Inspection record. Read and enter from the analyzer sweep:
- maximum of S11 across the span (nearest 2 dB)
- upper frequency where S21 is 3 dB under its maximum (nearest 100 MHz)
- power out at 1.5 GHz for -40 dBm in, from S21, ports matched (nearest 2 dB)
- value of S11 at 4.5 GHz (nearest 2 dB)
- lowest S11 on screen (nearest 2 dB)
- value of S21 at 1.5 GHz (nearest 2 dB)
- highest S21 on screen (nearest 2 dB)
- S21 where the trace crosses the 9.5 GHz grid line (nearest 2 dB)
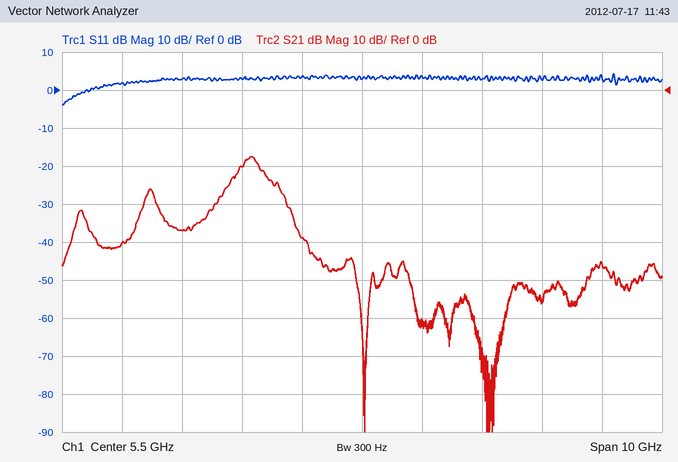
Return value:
4 dB
3.8 GHz
-80 dBm
4 dB
-4 dB
-40 dB
-18 dB
-46 dB
